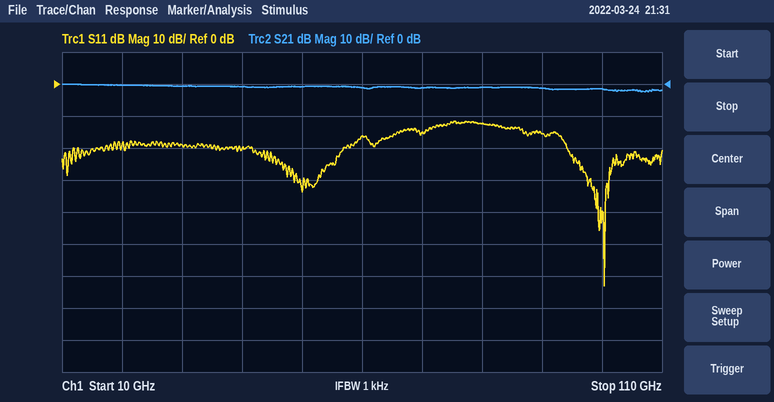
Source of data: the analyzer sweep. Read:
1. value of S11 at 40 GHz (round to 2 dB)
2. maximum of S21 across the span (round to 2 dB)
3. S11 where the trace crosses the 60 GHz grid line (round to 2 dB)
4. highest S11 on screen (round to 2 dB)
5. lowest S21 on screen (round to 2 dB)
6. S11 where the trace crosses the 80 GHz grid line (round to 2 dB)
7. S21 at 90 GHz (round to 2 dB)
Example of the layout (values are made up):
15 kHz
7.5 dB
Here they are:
-20 dB
0 dB
-16 dB
-12 dB
-2 dB
-12 dB
-2 dB
